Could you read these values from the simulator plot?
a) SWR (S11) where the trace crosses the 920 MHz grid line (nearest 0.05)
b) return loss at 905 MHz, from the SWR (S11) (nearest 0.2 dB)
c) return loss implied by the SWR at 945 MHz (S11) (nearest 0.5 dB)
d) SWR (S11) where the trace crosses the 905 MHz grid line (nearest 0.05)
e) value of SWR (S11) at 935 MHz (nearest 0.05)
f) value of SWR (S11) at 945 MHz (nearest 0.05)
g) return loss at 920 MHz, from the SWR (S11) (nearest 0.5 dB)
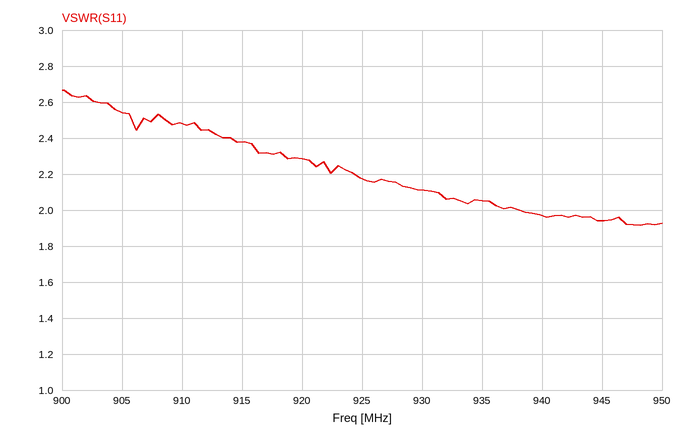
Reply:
2.30
7.2 dB
10.0 dB
2.55
2.05
1.95
8.0 dB
